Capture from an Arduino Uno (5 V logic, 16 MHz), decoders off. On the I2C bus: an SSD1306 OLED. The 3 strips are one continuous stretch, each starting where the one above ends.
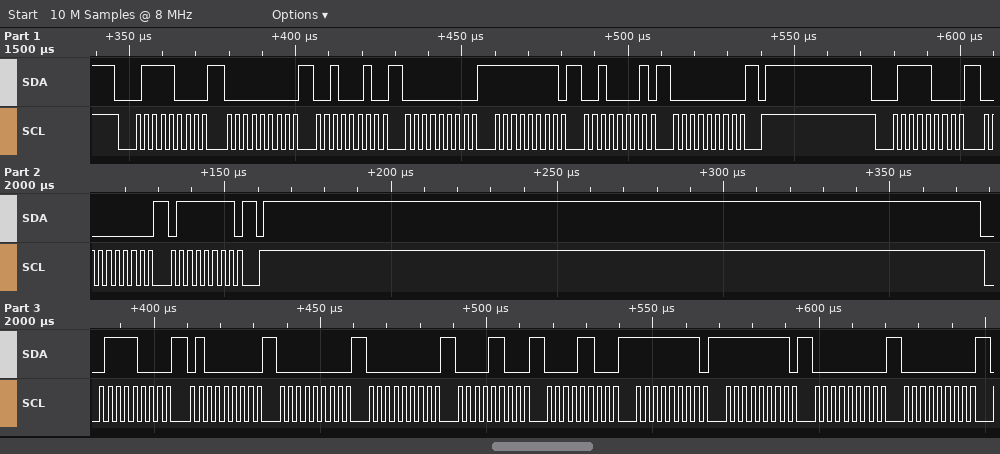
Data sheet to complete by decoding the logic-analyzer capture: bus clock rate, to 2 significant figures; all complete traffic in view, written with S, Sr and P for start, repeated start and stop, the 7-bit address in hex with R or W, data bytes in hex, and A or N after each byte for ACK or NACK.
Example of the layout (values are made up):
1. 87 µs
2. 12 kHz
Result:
1. 400 kHz
2. S 3CW A 00 A 22 A 00 A FF A 21 A 00 A P S 3CW A 00 A 7F A P S 3CW A 40 A 00 A 00 A 0C A 0C A FF A FF A 00 A 00 A
